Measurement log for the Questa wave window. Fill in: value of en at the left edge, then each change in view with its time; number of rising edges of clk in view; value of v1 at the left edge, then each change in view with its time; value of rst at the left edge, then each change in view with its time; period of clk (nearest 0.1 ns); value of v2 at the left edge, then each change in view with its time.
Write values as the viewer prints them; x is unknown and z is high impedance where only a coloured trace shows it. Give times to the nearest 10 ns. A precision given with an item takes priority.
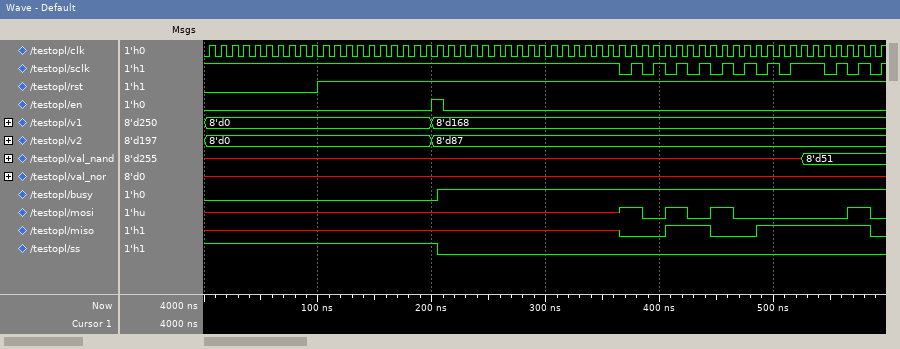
0, 1 at 200 ns, 0 at 210 ns
60
8'd0, 8'd168 at 200 ns
0, 1 at 100 ns
10 ns
8'd0, 8'd87 at 200 ns
